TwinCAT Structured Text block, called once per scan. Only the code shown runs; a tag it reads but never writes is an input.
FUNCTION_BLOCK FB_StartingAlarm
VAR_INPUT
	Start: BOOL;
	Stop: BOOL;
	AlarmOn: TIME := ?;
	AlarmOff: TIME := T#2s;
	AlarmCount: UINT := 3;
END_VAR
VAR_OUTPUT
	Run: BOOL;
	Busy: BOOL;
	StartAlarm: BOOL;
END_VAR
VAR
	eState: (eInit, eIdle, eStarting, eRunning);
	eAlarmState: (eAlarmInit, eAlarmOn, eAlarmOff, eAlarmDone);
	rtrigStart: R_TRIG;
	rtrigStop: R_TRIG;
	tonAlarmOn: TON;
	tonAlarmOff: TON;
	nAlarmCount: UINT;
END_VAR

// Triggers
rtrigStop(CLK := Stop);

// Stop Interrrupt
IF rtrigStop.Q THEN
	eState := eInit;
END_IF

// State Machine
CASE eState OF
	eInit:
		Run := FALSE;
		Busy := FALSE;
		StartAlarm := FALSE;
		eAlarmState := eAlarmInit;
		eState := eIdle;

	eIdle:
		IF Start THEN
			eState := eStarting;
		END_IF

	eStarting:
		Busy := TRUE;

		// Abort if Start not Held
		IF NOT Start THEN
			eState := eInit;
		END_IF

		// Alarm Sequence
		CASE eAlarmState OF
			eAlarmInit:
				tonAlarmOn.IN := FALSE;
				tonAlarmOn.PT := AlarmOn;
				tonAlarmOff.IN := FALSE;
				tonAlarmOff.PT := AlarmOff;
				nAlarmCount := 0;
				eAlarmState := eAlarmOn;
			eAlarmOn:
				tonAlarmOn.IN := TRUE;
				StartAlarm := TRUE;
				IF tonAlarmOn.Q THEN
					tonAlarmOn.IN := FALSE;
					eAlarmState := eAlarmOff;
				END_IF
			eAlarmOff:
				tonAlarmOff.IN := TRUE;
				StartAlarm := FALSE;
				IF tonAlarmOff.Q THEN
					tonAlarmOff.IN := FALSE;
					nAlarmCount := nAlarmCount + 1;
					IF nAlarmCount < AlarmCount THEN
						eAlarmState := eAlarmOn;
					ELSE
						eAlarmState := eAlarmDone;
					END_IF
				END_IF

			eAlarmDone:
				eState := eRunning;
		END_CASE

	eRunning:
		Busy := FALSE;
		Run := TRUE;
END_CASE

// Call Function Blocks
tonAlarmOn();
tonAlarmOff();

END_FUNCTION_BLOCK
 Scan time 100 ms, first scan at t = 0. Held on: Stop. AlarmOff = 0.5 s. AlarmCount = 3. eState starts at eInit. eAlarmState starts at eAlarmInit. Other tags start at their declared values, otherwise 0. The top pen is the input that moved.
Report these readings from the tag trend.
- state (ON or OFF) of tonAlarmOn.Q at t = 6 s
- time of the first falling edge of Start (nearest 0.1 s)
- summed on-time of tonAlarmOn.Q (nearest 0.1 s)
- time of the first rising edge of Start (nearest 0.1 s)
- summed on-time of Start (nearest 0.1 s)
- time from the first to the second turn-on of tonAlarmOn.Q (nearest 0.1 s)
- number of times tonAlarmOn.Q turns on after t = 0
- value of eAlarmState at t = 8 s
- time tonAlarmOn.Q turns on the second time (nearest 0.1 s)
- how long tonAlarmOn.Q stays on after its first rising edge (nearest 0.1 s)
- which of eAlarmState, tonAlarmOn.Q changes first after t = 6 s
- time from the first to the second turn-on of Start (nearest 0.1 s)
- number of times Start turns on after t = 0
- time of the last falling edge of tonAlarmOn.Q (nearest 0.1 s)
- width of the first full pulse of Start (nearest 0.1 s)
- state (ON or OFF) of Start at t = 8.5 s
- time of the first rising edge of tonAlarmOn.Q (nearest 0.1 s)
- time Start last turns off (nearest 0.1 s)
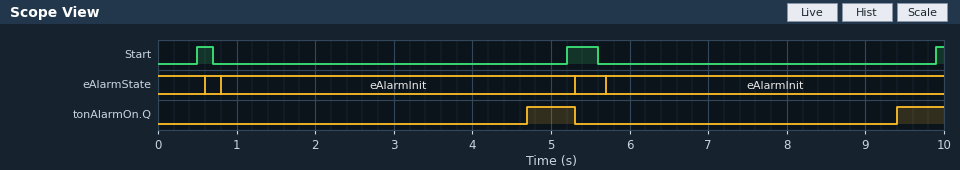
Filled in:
OFF
0.7 s
1.2 s
0.5 s
0.7 s
4.7 s
2
eAlarmInit
9.4 s
0.6 s
tonAlarmOn.Q
4.7 s
3
5.3 s
0.2 s
OFF
4.7 s
5.6 s
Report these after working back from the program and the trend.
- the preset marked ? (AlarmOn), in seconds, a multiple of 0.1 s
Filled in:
4.0 s
